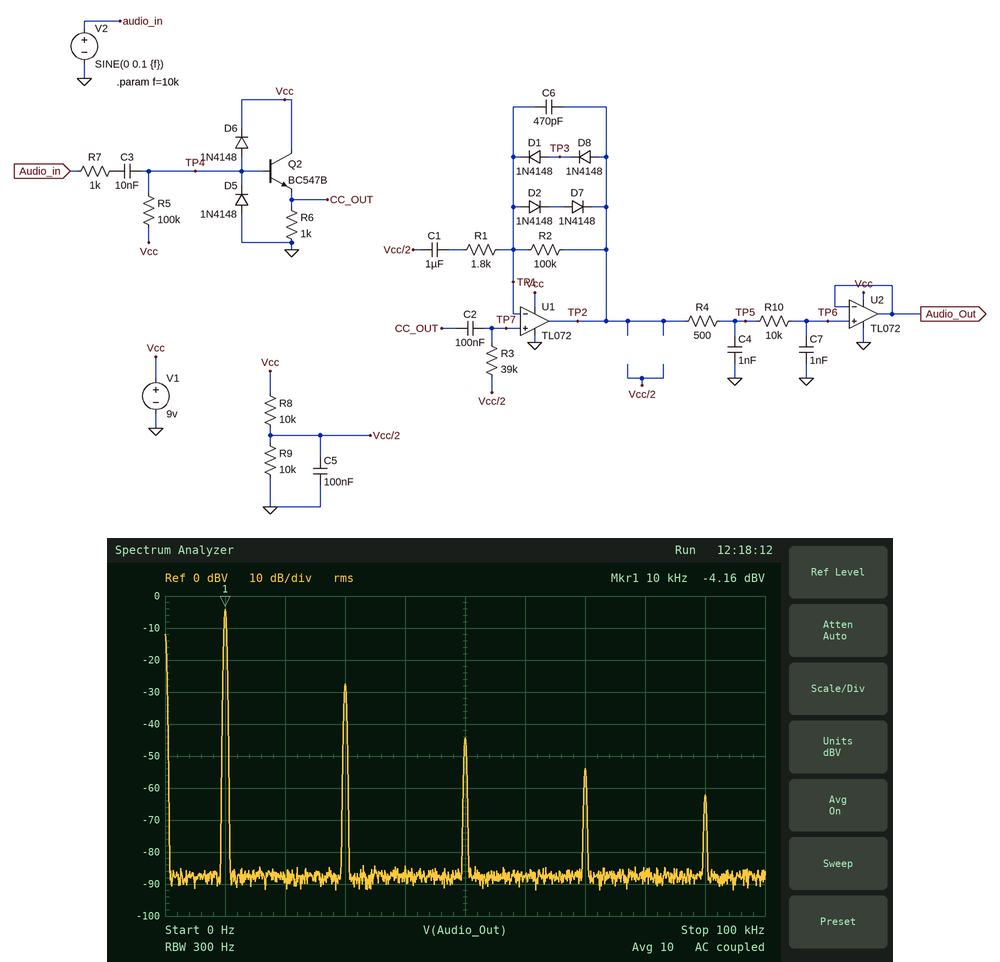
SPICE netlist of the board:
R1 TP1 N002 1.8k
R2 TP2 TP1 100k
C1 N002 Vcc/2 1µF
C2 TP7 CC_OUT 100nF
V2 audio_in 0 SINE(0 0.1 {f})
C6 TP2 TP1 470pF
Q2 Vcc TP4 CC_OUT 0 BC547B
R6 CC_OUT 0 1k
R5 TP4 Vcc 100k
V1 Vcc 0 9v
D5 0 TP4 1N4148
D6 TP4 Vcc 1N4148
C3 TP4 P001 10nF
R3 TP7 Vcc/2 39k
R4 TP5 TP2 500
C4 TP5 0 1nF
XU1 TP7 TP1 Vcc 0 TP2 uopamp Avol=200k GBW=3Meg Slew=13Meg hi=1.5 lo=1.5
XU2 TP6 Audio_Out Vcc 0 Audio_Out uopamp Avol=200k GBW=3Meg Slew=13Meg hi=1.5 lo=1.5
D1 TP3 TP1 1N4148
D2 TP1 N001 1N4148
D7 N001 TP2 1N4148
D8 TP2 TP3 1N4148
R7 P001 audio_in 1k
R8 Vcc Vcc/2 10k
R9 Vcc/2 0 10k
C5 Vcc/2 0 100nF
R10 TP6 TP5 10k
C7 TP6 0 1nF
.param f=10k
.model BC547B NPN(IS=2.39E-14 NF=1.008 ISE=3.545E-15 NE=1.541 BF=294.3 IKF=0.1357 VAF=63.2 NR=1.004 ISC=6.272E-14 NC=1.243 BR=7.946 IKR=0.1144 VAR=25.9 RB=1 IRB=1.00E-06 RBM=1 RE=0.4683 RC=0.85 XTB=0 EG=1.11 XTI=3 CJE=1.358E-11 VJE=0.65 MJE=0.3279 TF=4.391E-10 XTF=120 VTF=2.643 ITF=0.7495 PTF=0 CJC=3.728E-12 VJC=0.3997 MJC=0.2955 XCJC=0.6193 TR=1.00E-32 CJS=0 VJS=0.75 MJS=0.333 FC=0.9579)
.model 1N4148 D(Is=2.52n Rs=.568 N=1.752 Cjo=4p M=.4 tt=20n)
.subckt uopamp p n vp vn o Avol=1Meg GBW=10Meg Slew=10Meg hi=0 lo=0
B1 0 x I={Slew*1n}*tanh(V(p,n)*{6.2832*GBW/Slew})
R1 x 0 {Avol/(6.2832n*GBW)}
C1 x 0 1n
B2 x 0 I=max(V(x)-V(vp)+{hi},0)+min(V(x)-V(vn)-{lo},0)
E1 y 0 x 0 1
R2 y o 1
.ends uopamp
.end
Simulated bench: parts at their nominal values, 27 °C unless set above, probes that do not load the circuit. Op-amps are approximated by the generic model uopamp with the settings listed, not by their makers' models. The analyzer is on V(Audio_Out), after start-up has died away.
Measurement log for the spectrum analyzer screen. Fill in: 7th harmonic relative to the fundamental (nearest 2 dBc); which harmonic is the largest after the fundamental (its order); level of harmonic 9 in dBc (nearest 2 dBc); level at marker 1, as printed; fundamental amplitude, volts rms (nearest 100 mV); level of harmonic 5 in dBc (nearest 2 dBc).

-50 dBc
3
-58 dBc
-4.16 dBV
600 mV
-40 dBc
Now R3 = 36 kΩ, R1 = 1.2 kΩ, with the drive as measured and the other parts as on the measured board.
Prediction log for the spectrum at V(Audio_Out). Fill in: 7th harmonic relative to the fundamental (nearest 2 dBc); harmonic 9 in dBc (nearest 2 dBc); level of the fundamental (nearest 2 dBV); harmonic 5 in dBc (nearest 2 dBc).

-46 dBc
-54 dBc
-4 dBV
-36 dBc
